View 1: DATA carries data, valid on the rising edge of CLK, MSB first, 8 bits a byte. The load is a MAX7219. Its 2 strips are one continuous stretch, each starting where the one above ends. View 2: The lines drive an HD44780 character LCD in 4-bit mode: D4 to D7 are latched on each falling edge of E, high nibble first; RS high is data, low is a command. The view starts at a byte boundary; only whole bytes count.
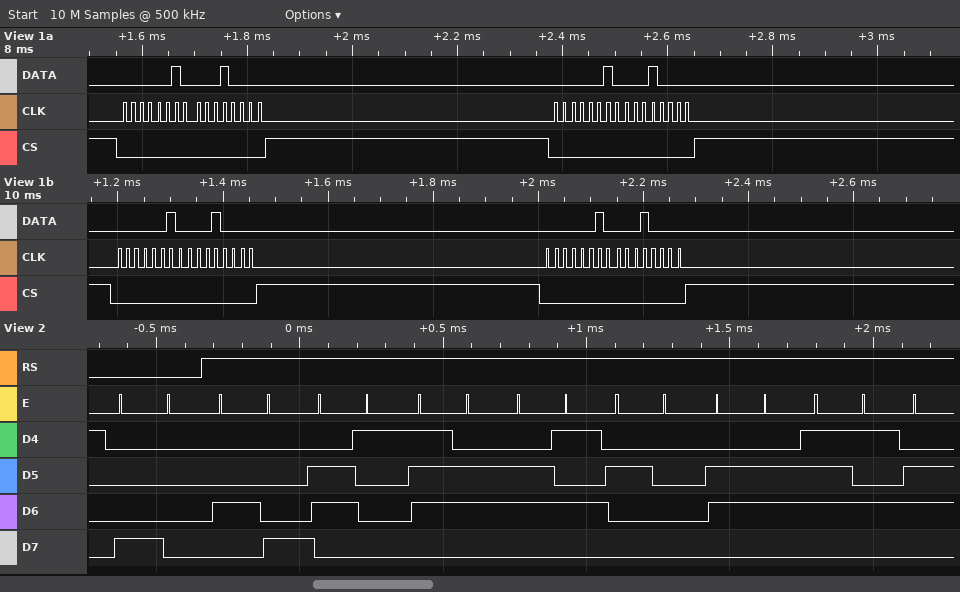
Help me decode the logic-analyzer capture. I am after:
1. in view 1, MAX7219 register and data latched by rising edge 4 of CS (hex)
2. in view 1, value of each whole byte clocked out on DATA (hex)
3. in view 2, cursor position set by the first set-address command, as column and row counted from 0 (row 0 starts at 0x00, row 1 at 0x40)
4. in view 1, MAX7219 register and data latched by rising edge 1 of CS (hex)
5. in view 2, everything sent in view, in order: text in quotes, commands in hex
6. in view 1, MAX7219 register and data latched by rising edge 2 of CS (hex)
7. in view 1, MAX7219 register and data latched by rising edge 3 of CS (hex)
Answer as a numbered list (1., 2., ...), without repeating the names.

1. register 0x2, data 0x10
2. 0x02 0x10 0x02 0x10 0x02 0x10 0x02 0x10
3. column 0, row 0
4. register 0x2, data 0x10
5. 0x80 "Have fu"
6. register 0x2, data 0x10
7. register 0x2, data 0x10
